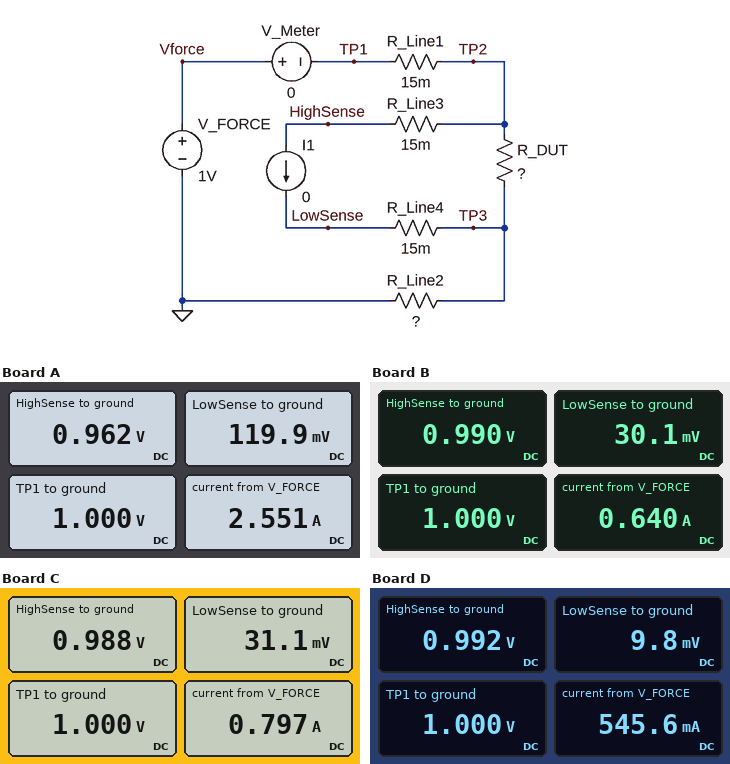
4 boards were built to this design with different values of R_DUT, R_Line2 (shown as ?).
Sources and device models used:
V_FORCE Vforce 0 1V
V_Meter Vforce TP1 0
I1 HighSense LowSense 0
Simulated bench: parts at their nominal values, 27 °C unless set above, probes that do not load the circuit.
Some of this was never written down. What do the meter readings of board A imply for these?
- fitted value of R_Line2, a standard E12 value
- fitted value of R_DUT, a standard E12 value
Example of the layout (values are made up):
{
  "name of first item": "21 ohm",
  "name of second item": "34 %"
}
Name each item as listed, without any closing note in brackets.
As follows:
{
  "fitted value of R_Line2, a standard E12 value": "0.047 Ω",
  "fitted value of R_DUT, a standard E12 value": "0.33 Ω"
}
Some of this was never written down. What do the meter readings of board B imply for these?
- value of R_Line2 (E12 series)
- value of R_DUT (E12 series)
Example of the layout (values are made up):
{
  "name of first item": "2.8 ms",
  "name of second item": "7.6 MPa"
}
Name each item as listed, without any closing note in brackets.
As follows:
{
  "value of R_Line2": "0.047 Ω",
  "value of R_DUT": "1.5 Ω"
}
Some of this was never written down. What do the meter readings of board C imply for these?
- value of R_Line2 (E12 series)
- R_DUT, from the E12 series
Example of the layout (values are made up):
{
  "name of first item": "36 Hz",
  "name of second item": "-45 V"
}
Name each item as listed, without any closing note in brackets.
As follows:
{
  "value of R_Line2": "0.039 Ω",
  "R_DUT, from the E12 series": "1.2 Ω"
}
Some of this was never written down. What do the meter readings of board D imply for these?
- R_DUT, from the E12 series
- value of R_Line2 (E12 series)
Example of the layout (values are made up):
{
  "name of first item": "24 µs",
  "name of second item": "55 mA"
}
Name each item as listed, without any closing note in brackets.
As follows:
{
  "R_DUT, from the E12 series": "1.8 Ω",
  "value of R_Line2": "0.018 Ω"
}
